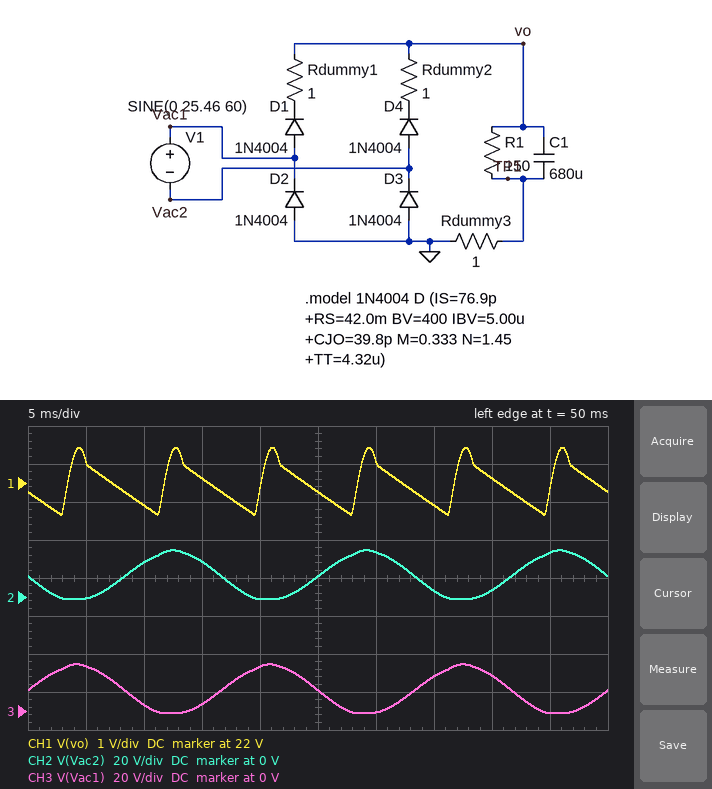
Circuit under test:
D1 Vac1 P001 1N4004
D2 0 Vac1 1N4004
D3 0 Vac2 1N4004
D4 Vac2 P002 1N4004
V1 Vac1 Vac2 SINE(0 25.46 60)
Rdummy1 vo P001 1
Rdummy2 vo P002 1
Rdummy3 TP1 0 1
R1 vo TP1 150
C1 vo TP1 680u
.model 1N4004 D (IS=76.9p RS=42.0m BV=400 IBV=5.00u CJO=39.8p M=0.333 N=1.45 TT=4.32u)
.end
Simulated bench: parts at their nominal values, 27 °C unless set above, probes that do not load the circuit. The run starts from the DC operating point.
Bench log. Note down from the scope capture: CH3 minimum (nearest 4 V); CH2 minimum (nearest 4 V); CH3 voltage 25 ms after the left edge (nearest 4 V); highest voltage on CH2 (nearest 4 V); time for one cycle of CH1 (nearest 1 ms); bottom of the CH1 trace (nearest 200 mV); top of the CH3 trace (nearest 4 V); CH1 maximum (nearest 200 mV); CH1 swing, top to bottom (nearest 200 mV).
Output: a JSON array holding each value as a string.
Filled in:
["0 V", "0 V", "12 V", "24 V", "8 ms", "21.2 V", "24 V", "23.0 V", "1.8 V"]
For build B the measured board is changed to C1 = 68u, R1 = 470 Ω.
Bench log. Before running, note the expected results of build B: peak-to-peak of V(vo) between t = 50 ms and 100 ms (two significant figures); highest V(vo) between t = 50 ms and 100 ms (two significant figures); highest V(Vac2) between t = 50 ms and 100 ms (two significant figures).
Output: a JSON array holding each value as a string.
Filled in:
["4.3 V", "24 V", "25 V"]
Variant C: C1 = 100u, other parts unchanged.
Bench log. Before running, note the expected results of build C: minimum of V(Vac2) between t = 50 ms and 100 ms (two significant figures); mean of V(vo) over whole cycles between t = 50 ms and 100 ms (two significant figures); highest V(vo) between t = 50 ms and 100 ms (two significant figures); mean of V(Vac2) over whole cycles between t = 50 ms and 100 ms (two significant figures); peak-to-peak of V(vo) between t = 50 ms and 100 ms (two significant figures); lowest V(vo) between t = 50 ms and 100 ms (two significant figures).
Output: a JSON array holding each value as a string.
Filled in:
["-880 mV", "20 V", "24 V", "10 V", "7.5 V", "16 V"]
